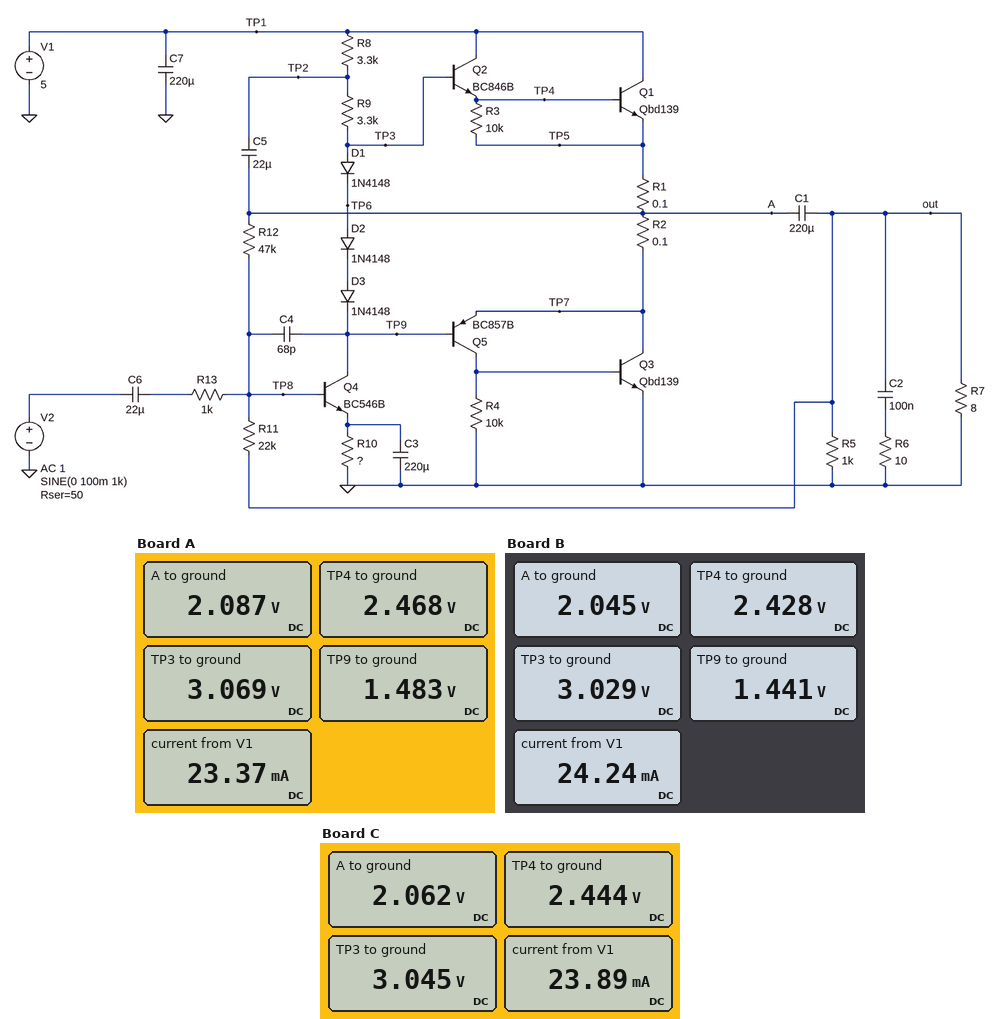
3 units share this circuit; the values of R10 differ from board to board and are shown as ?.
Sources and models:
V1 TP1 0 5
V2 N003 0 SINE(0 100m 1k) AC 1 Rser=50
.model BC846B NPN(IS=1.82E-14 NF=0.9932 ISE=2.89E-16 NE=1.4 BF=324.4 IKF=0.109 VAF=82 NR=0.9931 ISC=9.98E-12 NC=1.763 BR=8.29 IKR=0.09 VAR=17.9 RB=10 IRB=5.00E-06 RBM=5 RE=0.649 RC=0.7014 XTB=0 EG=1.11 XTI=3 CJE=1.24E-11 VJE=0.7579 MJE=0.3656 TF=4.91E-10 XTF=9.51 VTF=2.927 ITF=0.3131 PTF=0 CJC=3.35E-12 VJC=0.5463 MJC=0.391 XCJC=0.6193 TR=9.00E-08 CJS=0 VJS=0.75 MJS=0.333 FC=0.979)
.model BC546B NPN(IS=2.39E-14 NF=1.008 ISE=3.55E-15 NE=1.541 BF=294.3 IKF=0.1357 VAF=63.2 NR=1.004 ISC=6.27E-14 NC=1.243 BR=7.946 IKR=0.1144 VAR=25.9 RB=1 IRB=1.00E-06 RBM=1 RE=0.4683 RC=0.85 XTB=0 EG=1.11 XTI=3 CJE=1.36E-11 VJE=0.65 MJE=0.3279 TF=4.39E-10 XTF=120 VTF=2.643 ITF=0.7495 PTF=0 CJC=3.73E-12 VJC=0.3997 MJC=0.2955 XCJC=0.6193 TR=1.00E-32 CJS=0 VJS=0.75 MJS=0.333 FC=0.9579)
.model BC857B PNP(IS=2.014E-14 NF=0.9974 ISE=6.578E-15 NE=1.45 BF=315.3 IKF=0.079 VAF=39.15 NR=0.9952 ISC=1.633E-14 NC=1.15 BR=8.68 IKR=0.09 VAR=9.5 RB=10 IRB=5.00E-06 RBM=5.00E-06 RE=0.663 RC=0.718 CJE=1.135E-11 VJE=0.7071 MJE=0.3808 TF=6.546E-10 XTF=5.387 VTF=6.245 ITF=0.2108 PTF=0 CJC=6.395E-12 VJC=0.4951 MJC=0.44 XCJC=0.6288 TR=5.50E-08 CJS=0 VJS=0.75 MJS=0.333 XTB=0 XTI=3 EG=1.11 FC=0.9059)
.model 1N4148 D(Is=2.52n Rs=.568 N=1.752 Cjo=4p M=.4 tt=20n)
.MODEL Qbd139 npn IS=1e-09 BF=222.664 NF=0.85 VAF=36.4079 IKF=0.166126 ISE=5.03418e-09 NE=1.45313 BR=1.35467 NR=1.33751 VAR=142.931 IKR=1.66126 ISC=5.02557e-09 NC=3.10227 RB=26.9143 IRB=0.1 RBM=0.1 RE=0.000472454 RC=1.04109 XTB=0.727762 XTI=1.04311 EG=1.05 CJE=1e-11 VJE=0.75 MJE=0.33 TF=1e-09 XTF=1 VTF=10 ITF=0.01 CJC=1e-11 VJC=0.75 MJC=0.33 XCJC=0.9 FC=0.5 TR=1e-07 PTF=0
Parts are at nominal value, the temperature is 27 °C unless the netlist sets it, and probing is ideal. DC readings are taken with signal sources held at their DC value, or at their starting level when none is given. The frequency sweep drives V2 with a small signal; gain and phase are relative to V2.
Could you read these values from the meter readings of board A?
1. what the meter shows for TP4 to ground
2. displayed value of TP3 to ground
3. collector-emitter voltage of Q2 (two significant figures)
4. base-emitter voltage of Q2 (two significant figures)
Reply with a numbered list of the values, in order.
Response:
1. 2.468 V
2. 3.069 V
3. 2.5 V
4. 600 mV
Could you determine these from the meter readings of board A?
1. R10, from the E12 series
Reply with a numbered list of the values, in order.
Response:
1. 150 Ω
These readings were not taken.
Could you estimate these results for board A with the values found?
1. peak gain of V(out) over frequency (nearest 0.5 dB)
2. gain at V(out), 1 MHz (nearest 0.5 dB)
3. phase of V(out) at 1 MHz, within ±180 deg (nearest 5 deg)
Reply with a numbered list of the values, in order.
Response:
1. 22.5 dB
2. 4.5 dB
3. 85 deg
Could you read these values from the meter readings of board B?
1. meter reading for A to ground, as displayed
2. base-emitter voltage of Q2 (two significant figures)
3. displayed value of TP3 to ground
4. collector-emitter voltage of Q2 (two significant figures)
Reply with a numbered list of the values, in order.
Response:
1. 2.045 V
2. 600 mV
3. 3.029 V
4. 2.6 V
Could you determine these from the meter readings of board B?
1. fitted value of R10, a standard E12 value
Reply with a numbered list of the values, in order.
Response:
1. 100 Ω
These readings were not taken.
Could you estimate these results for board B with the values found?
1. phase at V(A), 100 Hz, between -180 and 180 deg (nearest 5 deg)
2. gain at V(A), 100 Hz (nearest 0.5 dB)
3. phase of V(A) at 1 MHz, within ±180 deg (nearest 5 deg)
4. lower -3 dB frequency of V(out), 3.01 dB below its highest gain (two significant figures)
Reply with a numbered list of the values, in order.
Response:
1. 160 deg
2. 25.0 dB
3. 85 deg
4. 29 Hz
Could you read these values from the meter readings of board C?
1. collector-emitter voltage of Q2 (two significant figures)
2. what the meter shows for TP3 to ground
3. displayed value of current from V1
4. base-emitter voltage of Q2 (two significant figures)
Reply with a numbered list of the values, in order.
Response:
1. 2.6 V
2. 3.045 V
3. 23.89 mA
4. 600 mV
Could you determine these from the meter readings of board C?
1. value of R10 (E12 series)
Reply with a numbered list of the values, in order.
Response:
1. 120 Ω
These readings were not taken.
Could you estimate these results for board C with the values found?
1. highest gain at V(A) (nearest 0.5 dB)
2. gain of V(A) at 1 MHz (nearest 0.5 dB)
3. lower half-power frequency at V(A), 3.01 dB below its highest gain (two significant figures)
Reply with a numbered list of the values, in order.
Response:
1. 31.0 dB
2. 4.5 dB
3. 7.4 Hz
